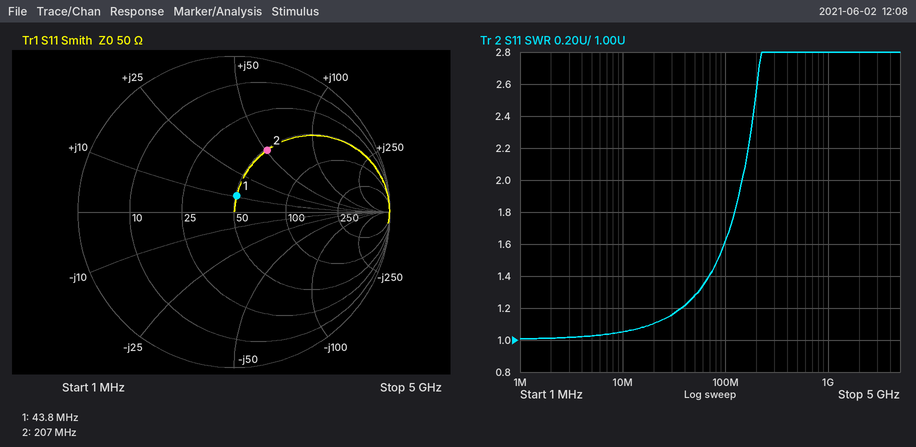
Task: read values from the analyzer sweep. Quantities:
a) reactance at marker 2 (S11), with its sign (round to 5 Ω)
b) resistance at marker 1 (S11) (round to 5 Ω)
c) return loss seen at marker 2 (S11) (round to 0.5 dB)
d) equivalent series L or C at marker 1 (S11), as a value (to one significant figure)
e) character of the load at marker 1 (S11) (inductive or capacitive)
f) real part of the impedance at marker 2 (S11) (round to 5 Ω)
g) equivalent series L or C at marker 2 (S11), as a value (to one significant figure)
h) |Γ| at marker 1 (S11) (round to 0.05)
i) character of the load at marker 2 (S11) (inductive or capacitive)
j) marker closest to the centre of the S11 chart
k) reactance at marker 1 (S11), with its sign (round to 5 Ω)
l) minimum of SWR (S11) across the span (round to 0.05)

+50 Ω
50 Ω
7.0 dB
40 nH
inductive
50 Ω
40 nH
0.10
inductive
marker 1
+10 Ω
1.00
